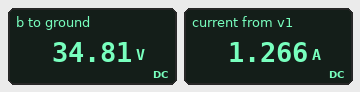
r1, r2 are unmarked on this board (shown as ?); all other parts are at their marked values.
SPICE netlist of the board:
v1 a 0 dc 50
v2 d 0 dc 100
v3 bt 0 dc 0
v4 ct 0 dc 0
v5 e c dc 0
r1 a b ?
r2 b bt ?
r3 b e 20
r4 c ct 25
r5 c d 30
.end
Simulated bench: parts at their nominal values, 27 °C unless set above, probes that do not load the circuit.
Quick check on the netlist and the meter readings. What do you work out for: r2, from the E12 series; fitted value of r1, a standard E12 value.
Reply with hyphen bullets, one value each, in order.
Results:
- 22 Ω
- 12 Ω
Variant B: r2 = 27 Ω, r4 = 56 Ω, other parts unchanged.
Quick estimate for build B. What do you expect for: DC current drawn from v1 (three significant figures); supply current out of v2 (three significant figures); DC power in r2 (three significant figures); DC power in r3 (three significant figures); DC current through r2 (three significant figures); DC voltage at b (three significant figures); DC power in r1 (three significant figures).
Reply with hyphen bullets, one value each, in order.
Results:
- 841 mA
- 1.58 A
- 59.0 W
- 8.13 W
- 1.48 A
- 39.9 V
- 8.48 W
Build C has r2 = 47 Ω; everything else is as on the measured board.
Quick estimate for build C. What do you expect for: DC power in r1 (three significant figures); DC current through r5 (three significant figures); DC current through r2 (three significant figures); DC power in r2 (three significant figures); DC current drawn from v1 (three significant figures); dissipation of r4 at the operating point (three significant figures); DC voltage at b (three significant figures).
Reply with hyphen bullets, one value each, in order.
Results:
- 6.64 W
- 1.88 A
- 874 mA
- 35.9 W
- 744 mA
- 76.3 W
- 41.1 V
